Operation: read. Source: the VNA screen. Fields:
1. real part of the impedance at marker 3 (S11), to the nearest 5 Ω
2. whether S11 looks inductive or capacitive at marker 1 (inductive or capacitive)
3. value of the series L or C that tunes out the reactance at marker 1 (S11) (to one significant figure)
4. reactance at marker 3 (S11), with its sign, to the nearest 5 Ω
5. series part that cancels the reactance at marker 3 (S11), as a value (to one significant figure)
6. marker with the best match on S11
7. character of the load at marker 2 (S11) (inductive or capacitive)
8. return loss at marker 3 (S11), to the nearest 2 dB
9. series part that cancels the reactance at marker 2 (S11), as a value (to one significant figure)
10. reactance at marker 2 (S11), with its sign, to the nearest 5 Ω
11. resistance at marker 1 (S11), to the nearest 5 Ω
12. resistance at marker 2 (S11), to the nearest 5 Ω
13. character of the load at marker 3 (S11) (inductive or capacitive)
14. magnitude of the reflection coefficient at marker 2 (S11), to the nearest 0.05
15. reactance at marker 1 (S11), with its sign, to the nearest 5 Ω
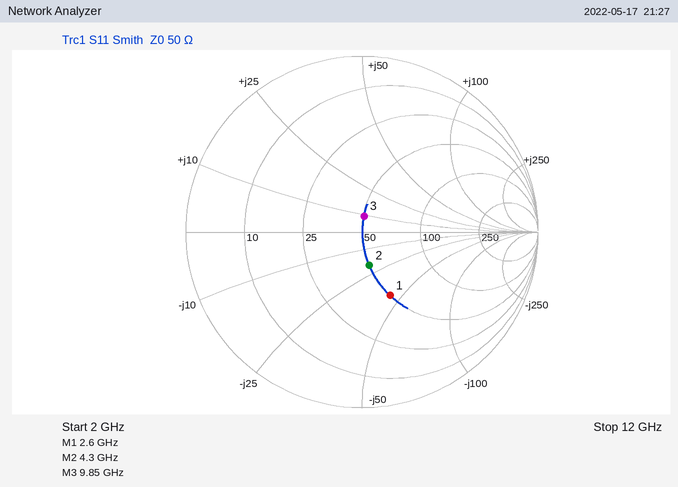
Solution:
50 Ω
capacitive
3 nH
+10 Ω
2 pF
marker 3
capacitive
20 dB
700 pH
-20 Ω
50 Ω
50 Ω
inductive
0.20
-45 Ω
